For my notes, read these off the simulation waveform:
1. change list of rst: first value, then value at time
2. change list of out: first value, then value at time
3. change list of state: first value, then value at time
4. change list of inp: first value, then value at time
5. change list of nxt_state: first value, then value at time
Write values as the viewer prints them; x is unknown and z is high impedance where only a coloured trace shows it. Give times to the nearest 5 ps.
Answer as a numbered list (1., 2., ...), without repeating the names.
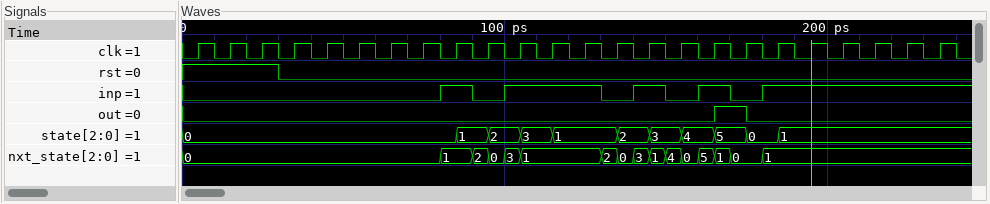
1. 1, 0 at 30 ps
2. 0, 1 at 165 ps, 0 at 175 ps
3. 0, 1 at 85 ps, 2 at 95 ps, 3 at 105 ps, 1 at 115 ps, 2 at 135 ps, 3 at 145 ps, 4 at 155 ps, 5 at 165 ps, 0 at 175 ps, 1 at 185 ps
4. 0, 1 at 80 ps, 0 at 90 ps, 1 at 100 ps, 0 at 130 ps, 1 at 140 ps, 0 at 150 ps, 1 at 160 ps, 0 at 170 ps, 1 at 180 ps
5. 0, 1 at 80 ps, 2 at 90 ps, 0 at 95 ps, 3 at 100 ps, 1 at 105 ps, 2 at 130 ps, 0 at 135 ps, 3 at 140 ps, 1 at 145 ps, 4 at 150 ps, 0 at 155 ps, 5 at 160 ps, 1 at 165 ps, 0 at 170 ps, 1 at 180 ps
